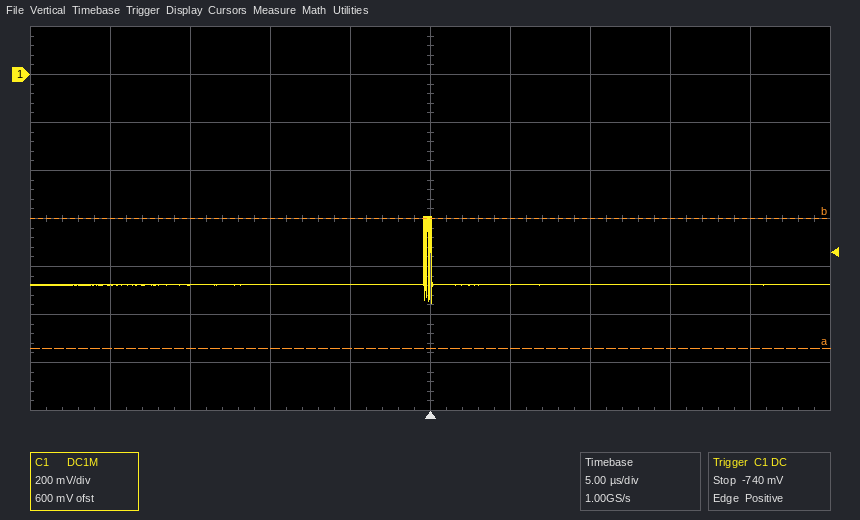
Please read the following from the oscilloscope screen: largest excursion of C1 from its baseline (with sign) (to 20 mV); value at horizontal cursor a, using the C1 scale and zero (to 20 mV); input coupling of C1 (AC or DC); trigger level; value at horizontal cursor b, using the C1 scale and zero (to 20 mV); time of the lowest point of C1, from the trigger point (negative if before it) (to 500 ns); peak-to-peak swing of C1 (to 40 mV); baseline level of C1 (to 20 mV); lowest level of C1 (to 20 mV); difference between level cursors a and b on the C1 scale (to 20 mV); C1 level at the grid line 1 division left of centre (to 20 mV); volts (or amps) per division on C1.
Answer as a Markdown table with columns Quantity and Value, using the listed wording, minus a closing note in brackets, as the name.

| Quantity | Value |
|---|---|
| largest excursion of C1 from its baseline (with sign) | +280 mV |
| value at horizontal cursor a, using the C1 scale and zero | -1.14 V |
| input coupling of C1 | DC |
| trigger level | -740 mV |
| value at horizontal cursor b, using the C1 scale and zero | -600 mV |
| time of the lowest point of C1, from the trigger point (negative if before it) | 0.0 µs |
| peak-to-peak swing of C1 | 360 mV |
| baseline level of C1 | -880 mV |
| lowest level of C1 | -960 mV |
| difference between level cursors a and b on the C1 scale | 540 mV |
| C1 level at the grid line 1 division left of centre | -880 mV |
| volts (or amps) per division on C1 | 200 mV |
